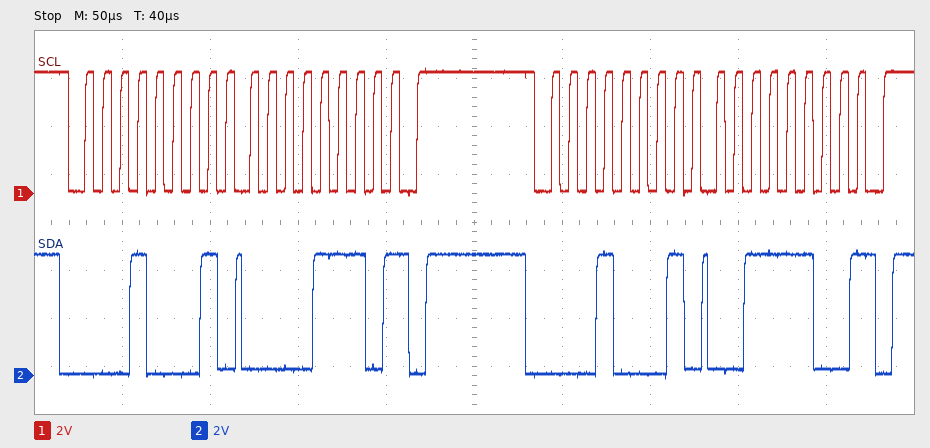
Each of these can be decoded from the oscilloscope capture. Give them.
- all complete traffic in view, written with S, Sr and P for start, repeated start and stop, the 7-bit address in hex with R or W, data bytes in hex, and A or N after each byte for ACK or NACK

S 08R A 0E N P S 08R A 3C N P
